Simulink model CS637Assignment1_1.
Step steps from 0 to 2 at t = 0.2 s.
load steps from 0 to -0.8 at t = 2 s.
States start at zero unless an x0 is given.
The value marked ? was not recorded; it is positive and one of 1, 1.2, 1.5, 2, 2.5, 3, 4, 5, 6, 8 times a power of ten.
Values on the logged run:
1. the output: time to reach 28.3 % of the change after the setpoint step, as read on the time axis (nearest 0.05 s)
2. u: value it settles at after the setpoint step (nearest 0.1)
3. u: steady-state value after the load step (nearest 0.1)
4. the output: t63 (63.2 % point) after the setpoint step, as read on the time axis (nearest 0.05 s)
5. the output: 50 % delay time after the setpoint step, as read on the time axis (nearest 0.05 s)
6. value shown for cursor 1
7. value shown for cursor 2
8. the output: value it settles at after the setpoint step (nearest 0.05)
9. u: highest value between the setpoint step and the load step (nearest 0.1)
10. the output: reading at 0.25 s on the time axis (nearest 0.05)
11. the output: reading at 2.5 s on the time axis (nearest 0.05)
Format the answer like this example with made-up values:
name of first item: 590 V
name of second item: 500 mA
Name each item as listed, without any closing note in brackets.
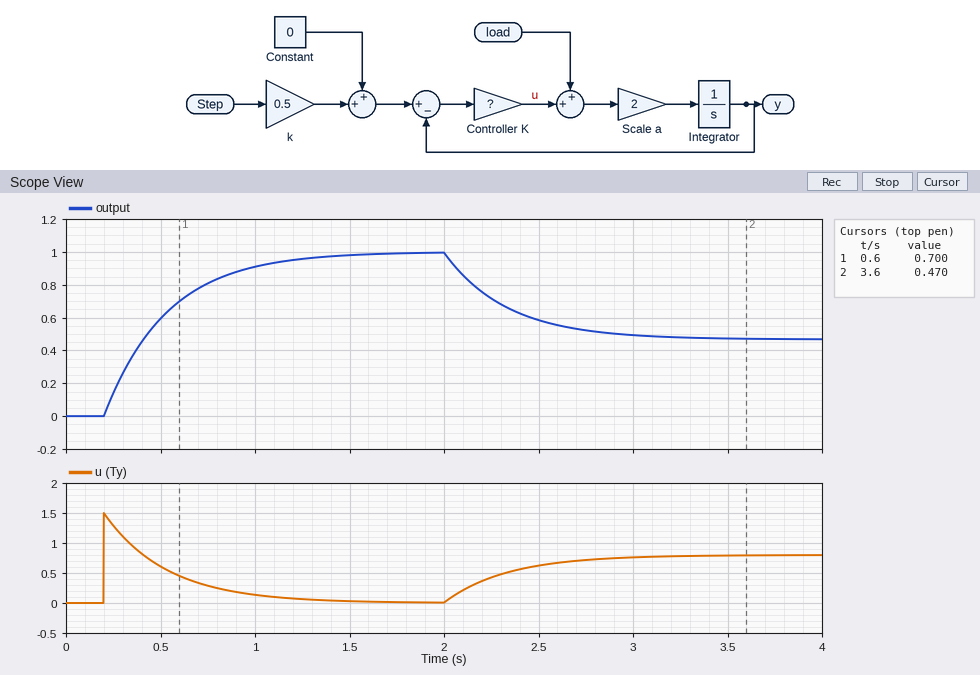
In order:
the output: time to reach 28.3 % of the change after the setpoint step, as read on the time axis: 0.30 s
u: value it settles at after the setpoint step: 0.0
u: steady-state value after the load step: 0.8
the output: t63 (63.2 % point) after the setpoint step, as read on the time axis: 0.55 s
the output: 50 % delay time after the setpoint step, as read on the time axis: 0.45 s
value shown for cursor 1: 0.700
value shown for cursor 2: 0.470
the output: value it settles at after the setpoint step: 1.00
u: highest value between the setpoint step and the load step: 1.5
the output: reading at 0.25 s on the time axis: 0.15
the output: reading at 2.5 s on the time axis: 0.60
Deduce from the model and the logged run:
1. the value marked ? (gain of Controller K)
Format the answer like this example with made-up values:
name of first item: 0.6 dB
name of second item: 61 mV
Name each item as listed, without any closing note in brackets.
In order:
the value marked ?: 1.5
